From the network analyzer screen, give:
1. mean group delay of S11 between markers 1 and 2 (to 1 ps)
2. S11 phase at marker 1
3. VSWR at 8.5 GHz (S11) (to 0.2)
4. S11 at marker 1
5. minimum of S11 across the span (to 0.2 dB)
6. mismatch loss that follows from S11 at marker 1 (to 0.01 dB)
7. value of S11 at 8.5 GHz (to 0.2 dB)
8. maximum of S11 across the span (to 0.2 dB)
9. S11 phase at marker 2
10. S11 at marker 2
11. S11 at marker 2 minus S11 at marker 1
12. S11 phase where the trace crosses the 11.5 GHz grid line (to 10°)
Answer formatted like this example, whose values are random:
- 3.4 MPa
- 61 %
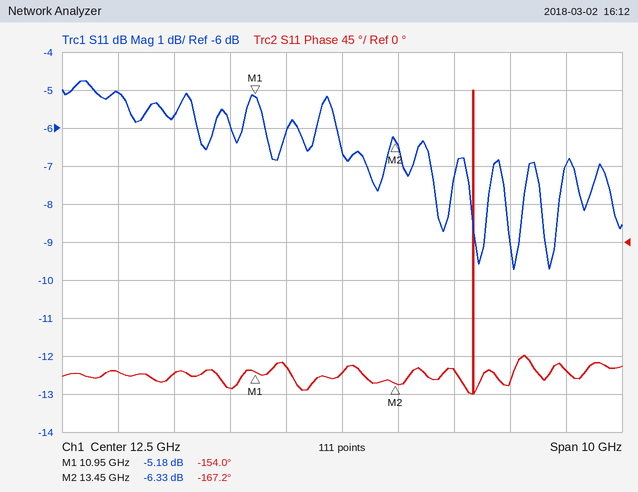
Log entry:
- 15 ps
- -154.0°
- 3.6
- -5.18 dB
- -9.8 dB
- 1.57 dB
- -5.0 dB
- -4.8 dB
- -167.2°
- -6.33 dB
- -1.15 dB
- -150°
